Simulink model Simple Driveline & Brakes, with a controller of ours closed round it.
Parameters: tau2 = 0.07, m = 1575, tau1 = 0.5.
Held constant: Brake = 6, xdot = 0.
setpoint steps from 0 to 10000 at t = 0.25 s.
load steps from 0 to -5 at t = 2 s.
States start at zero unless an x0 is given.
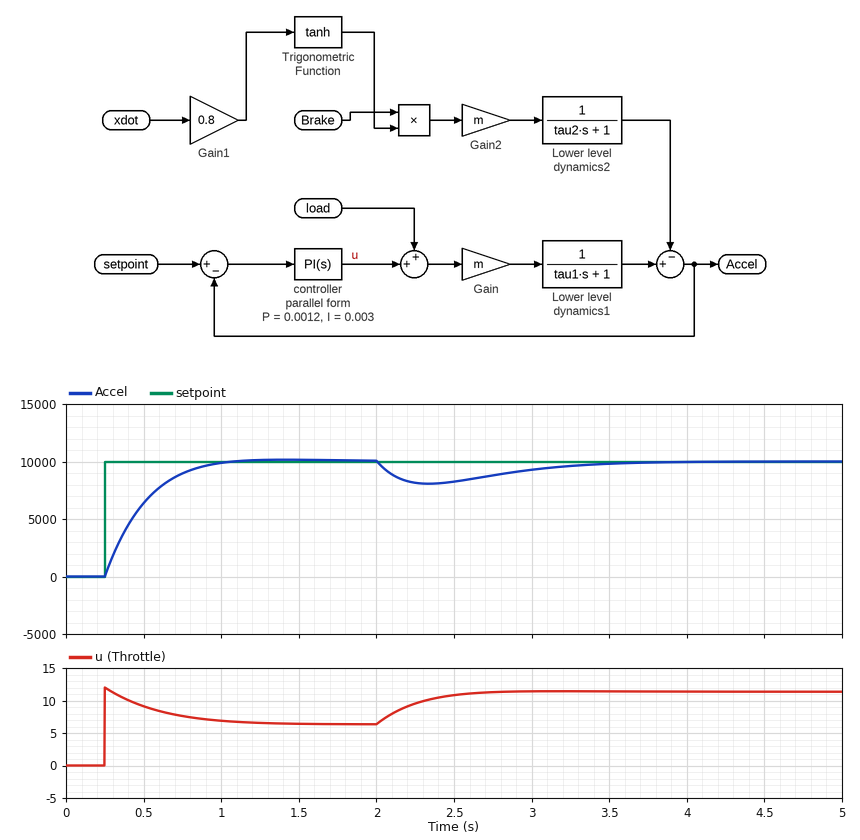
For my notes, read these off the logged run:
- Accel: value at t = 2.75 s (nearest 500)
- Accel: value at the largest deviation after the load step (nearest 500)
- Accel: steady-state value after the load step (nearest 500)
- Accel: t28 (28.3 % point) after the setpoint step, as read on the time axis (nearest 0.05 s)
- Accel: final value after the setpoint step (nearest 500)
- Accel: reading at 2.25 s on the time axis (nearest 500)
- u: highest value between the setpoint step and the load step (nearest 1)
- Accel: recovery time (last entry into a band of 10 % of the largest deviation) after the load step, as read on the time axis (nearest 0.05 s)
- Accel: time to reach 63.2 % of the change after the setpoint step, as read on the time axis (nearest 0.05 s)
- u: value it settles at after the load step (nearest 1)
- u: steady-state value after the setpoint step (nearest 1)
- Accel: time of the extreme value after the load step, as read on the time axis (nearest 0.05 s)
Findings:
9000
8000
10000
0.35 s
10000
8000
12
3.50 s
0.50 s
11
6
2.35 s
